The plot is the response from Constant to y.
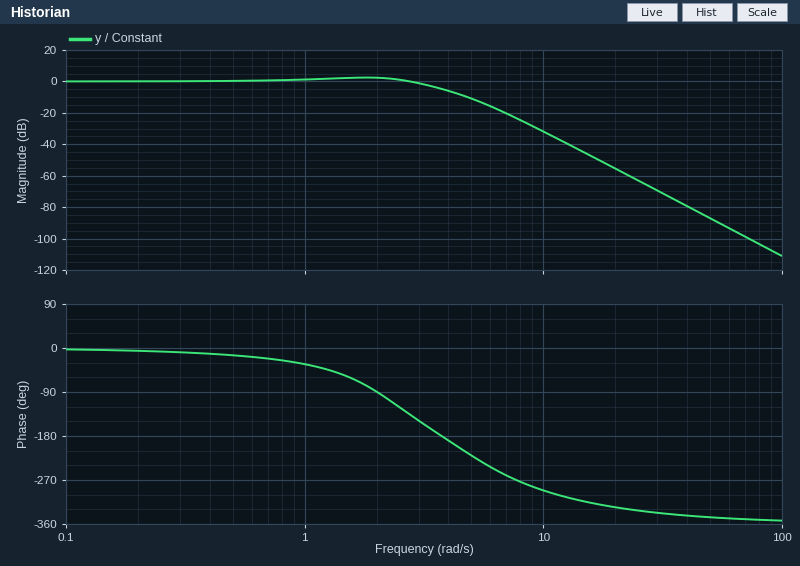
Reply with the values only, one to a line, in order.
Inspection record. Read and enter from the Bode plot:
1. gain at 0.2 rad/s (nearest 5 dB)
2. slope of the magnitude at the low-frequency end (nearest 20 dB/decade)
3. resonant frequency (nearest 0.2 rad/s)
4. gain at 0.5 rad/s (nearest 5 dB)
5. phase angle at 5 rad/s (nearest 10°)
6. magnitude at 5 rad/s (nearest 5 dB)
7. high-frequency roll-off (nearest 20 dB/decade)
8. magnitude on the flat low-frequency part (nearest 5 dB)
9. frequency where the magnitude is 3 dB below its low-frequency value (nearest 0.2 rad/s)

0 dB
0 dB/decade
1.8 rad/s
0 dB
-220°
-10 dB
-80 dB/decade
0 dB
3.4 rad/s
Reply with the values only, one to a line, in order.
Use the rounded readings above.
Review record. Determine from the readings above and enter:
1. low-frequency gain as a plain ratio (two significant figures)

1.0
